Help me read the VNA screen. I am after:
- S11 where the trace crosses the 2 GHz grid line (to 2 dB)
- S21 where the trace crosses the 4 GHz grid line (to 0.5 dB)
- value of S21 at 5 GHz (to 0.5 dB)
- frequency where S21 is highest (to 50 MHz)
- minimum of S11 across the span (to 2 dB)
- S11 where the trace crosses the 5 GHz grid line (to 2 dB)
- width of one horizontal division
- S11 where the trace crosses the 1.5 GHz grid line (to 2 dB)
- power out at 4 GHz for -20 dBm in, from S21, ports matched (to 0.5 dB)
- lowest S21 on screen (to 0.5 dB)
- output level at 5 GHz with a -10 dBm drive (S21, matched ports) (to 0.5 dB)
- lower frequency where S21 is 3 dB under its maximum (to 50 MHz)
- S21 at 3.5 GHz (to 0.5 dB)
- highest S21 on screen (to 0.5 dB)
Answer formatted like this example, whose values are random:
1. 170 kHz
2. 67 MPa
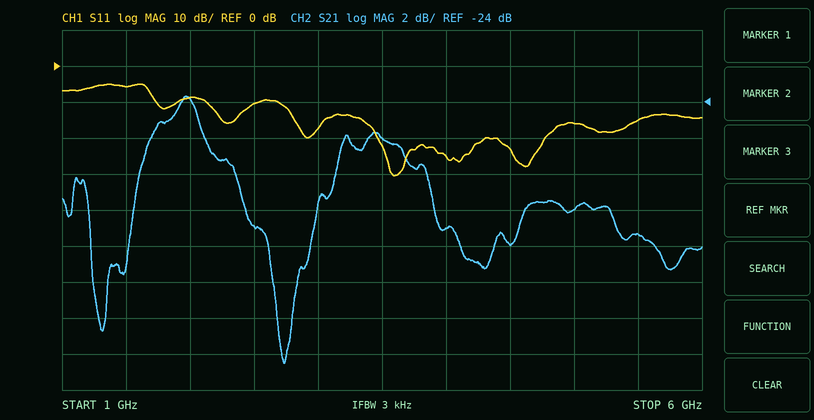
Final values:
1. -8 dB
2. -31.0 dB
3. -30.0 dB
4. 1.95 GHz
5. -30 dB
6. -16 dB
7. 500 MHz
8. -6 dB
9. -51.0 dBm
10. -38.5 dB
11. -40.0 dBm
12. 1.65 GHz
13. -26.0 dB
14. -23.5 dB
